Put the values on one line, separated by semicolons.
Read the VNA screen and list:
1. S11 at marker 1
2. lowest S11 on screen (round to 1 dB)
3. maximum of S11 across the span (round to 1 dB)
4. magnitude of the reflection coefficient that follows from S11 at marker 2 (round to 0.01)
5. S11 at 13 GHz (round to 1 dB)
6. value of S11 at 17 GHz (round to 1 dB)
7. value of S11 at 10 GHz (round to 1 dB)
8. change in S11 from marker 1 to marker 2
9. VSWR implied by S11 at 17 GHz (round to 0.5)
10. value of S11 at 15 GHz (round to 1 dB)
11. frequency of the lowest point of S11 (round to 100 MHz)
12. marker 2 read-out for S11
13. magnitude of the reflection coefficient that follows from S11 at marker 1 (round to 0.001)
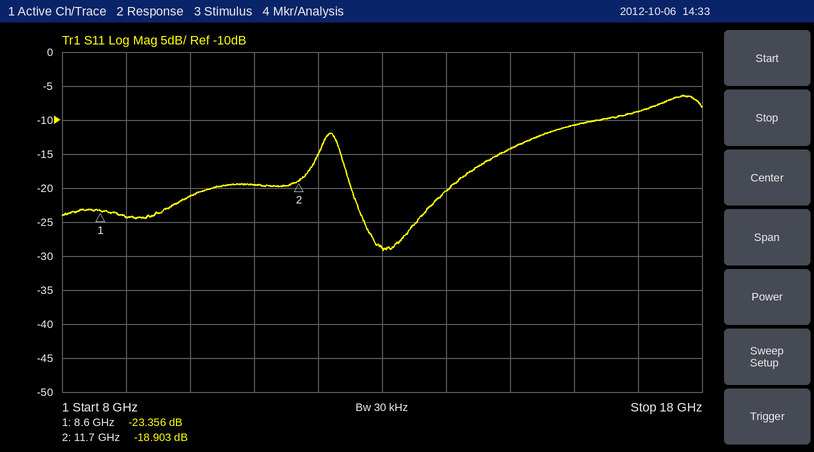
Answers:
-23.356 dB; -29 dB; -6 dB; 0.11; -29 dB; -9 dB; -21 dB; 4.453 dB; 2.0; -14 dB; 13.0 GHz; -18.903 dB; 0.068
